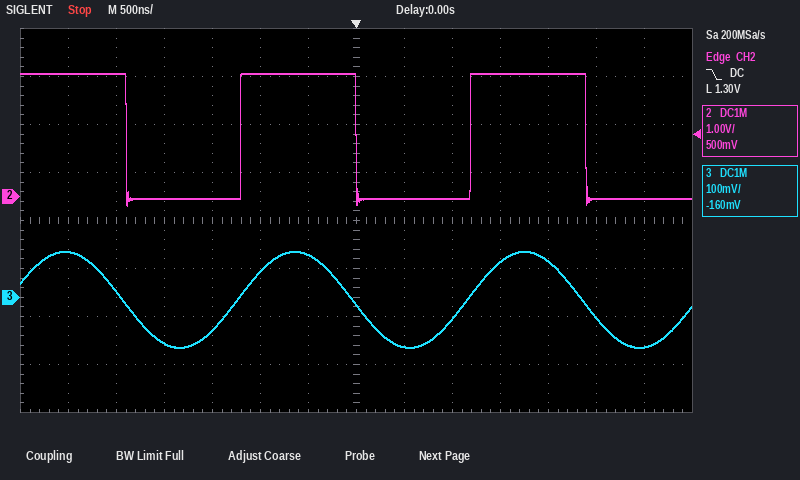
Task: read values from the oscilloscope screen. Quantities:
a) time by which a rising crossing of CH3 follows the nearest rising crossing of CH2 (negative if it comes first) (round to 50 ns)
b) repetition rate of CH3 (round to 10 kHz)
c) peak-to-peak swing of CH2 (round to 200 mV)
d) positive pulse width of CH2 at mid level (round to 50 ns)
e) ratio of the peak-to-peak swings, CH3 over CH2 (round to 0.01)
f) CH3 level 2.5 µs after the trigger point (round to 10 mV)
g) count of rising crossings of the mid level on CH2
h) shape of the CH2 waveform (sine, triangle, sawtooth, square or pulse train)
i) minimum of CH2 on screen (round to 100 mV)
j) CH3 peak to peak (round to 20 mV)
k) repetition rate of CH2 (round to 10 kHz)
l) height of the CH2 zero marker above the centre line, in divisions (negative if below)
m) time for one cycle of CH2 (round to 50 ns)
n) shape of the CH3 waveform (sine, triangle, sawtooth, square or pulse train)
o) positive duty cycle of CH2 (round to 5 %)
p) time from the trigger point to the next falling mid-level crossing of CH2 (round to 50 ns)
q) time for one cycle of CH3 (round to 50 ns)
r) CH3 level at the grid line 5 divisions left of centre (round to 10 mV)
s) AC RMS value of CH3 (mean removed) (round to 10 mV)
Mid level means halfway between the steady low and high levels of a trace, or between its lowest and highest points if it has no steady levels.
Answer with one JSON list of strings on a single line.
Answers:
["-50 ns", "420 kHz", "2.8 V", "1.20 µs", "0.07", "-40 mV", "2", "square", "-200 mV", "200 mV", "420 kHz", "+0.5 div", "2.40 µs", "sine", "50 %", "2.40 µs", "2.40 µs", "10 mV", "70 mV"]
